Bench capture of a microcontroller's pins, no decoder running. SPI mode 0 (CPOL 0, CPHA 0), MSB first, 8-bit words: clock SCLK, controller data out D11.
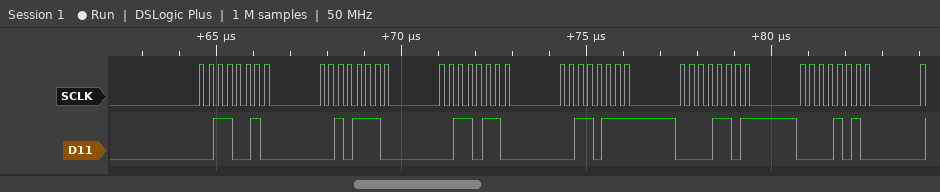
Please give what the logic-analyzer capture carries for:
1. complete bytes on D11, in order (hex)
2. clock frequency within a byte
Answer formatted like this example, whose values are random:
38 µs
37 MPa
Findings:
0x32 0x2E 0x36 0x37 0x0D 0x0A
4 MHz
